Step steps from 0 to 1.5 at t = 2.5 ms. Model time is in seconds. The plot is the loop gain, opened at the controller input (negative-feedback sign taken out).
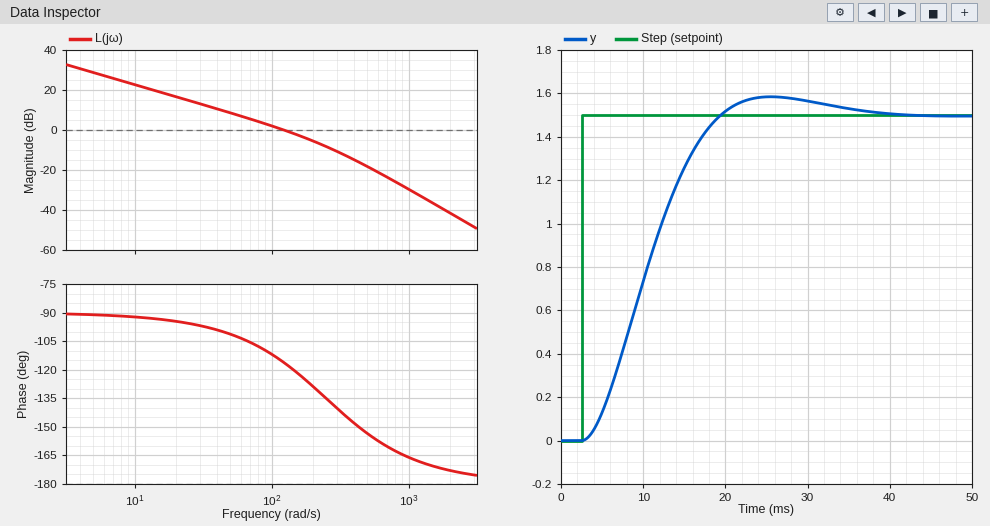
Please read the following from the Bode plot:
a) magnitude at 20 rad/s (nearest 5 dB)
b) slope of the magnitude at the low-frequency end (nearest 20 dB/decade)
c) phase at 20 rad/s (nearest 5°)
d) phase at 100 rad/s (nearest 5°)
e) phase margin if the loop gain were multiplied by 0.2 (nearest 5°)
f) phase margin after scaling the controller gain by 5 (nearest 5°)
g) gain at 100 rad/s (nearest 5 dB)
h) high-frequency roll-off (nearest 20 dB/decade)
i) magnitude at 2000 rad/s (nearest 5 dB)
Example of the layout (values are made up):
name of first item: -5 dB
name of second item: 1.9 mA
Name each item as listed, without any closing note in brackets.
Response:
magnitude at 20 rad/s: 15 dB
slope of the magnitude at the low-frequency end: -20 dB/decade
phase at 20 rad/s: -95°
phase at 100 rad/s: -110°
phase margin if the loop gain were multiplied by 0.2: 85°
phase margin after scaling the controller gain by 5: 35°
gain at 100 rad/s: 0 dB
high-frequency roll-off: -40 dB/decade
magnitude at 2000 rad/s: -40 dB
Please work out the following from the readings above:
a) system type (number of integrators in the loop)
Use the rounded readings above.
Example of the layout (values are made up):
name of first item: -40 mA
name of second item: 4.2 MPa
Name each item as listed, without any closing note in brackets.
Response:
system type: 1
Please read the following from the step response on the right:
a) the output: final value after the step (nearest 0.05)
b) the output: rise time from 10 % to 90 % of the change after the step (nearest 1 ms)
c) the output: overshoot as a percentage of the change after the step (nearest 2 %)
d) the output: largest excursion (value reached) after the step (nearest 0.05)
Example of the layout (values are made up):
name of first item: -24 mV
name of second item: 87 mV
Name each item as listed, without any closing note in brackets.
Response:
the output: final value after the step: 1.50
the output: rise time from 10 % to 90 % of the change after the step: 11 ms
the output: overshoot as a percentage of the change after the step: 6 %
the output: largest excursion (value reached) after the step: 1.60
